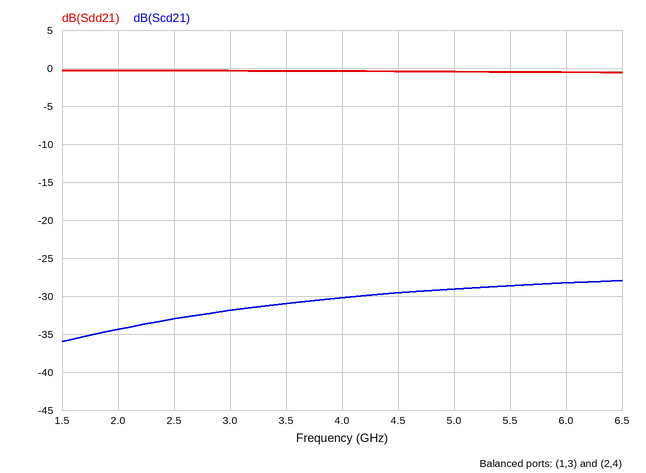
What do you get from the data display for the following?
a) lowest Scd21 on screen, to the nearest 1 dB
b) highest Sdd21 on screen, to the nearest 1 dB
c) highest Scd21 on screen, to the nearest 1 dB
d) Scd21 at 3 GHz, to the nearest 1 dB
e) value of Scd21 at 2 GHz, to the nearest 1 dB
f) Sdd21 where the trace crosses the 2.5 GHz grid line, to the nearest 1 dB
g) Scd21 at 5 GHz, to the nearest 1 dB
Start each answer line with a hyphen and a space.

- -36 dB
- 0 dB
- -28 dB
- -32 dB
- -34 dB
- 0 dB
- -29 dB
